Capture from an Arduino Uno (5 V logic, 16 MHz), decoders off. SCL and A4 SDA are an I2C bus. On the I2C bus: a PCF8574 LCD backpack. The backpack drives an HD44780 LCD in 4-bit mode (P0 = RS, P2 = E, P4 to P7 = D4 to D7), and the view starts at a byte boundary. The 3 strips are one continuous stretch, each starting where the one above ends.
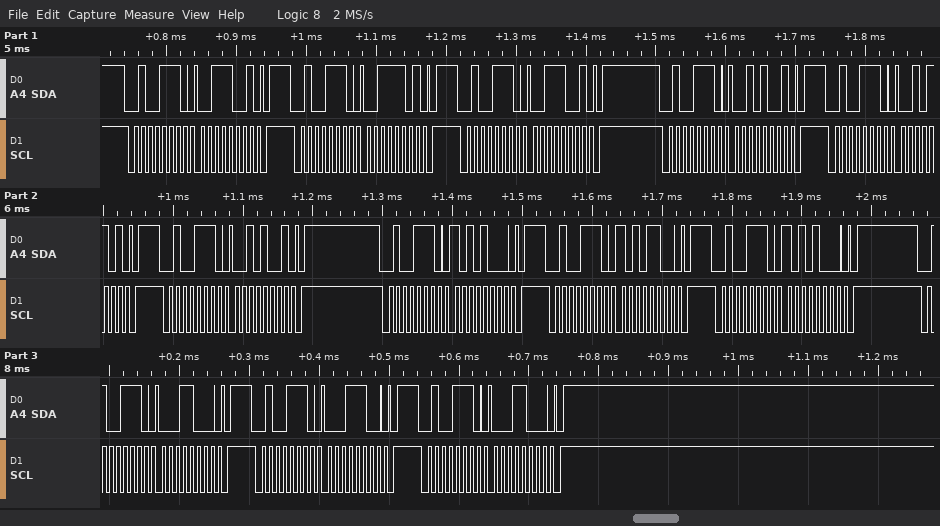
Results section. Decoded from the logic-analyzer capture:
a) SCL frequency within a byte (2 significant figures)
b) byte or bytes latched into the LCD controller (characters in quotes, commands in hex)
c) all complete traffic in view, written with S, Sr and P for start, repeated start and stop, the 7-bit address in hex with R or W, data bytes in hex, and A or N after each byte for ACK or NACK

100 kHz
'2' 0xA1
S 27W A 39 A P S 27W A 3D A P S 27W A 39 A P S 27W A 29 A P S 27W A 2D A P S 27W A 29 A P S 27W A A8 A P S 27W A AC A P S 27W A A8 A P S 27W A 18 A P S 27W A 1C A P S 27W A 18 A P
